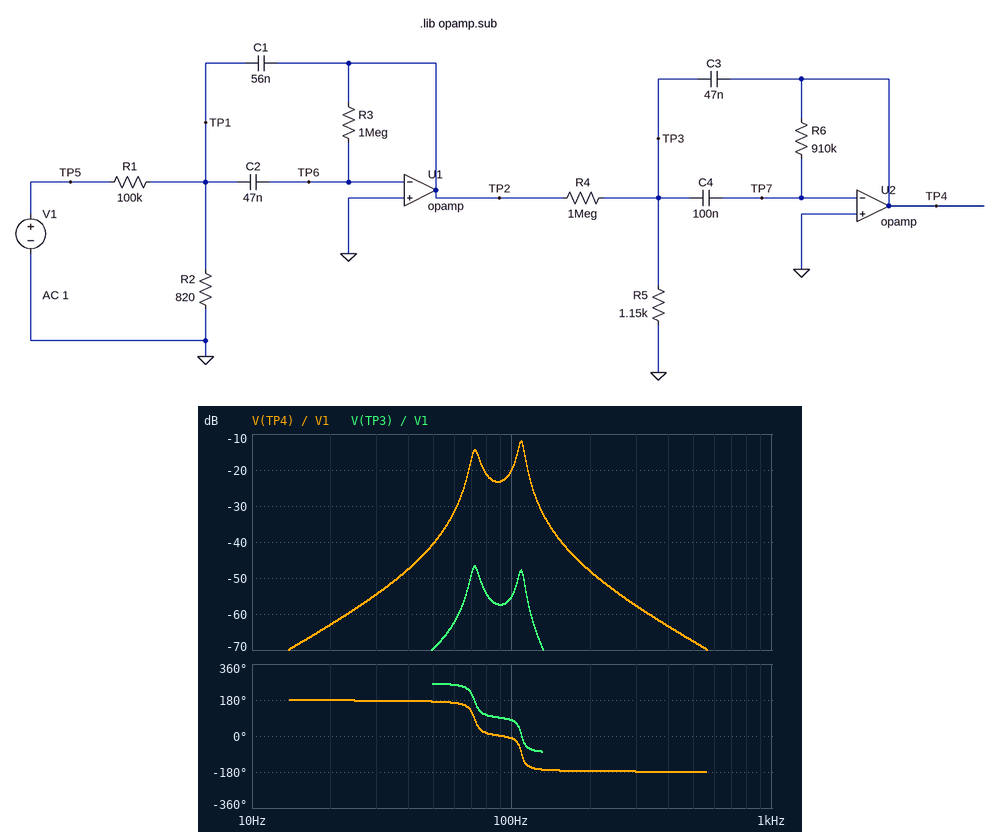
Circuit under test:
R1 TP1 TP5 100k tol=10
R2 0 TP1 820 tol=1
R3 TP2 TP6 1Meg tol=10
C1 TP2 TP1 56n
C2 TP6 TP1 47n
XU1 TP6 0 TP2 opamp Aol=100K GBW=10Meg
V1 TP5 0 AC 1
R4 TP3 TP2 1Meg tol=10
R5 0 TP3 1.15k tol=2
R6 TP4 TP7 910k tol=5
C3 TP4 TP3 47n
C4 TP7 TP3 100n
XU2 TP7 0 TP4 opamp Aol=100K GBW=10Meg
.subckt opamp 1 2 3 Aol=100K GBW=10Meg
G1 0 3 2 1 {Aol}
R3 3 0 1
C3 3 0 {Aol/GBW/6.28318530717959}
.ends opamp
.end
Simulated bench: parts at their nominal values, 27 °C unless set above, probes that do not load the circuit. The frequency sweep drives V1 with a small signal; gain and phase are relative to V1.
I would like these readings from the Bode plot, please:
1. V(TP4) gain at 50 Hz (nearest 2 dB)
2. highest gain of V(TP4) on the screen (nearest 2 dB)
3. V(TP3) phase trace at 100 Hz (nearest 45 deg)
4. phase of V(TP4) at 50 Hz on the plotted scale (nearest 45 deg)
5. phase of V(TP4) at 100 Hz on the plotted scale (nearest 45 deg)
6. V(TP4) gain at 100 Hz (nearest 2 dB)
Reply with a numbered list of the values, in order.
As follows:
1. -40 dB
2. -12 dB
3. 90 deg
4. 180 deg
5. 0 deg
6. -20 dB
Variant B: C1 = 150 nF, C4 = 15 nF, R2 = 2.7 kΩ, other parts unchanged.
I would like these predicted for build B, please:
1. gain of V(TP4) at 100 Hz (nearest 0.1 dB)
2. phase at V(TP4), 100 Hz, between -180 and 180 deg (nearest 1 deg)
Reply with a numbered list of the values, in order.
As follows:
1. -55.4 dB
2. -1 deg
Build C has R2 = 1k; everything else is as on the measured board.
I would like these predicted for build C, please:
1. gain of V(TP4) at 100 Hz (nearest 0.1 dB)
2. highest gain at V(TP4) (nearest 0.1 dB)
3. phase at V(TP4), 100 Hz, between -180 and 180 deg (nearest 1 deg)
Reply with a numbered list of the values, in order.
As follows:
1. -10.8 dB
2. -9.6 dB
3. -108 deg
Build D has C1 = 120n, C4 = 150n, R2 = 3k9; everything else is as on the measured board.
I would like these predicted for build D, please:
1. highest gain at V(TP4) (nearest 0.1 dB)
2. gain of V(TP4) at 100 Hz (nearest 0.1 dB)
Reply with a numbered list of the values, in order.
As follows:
1. -12.5 dB
2. -42.2 dB
